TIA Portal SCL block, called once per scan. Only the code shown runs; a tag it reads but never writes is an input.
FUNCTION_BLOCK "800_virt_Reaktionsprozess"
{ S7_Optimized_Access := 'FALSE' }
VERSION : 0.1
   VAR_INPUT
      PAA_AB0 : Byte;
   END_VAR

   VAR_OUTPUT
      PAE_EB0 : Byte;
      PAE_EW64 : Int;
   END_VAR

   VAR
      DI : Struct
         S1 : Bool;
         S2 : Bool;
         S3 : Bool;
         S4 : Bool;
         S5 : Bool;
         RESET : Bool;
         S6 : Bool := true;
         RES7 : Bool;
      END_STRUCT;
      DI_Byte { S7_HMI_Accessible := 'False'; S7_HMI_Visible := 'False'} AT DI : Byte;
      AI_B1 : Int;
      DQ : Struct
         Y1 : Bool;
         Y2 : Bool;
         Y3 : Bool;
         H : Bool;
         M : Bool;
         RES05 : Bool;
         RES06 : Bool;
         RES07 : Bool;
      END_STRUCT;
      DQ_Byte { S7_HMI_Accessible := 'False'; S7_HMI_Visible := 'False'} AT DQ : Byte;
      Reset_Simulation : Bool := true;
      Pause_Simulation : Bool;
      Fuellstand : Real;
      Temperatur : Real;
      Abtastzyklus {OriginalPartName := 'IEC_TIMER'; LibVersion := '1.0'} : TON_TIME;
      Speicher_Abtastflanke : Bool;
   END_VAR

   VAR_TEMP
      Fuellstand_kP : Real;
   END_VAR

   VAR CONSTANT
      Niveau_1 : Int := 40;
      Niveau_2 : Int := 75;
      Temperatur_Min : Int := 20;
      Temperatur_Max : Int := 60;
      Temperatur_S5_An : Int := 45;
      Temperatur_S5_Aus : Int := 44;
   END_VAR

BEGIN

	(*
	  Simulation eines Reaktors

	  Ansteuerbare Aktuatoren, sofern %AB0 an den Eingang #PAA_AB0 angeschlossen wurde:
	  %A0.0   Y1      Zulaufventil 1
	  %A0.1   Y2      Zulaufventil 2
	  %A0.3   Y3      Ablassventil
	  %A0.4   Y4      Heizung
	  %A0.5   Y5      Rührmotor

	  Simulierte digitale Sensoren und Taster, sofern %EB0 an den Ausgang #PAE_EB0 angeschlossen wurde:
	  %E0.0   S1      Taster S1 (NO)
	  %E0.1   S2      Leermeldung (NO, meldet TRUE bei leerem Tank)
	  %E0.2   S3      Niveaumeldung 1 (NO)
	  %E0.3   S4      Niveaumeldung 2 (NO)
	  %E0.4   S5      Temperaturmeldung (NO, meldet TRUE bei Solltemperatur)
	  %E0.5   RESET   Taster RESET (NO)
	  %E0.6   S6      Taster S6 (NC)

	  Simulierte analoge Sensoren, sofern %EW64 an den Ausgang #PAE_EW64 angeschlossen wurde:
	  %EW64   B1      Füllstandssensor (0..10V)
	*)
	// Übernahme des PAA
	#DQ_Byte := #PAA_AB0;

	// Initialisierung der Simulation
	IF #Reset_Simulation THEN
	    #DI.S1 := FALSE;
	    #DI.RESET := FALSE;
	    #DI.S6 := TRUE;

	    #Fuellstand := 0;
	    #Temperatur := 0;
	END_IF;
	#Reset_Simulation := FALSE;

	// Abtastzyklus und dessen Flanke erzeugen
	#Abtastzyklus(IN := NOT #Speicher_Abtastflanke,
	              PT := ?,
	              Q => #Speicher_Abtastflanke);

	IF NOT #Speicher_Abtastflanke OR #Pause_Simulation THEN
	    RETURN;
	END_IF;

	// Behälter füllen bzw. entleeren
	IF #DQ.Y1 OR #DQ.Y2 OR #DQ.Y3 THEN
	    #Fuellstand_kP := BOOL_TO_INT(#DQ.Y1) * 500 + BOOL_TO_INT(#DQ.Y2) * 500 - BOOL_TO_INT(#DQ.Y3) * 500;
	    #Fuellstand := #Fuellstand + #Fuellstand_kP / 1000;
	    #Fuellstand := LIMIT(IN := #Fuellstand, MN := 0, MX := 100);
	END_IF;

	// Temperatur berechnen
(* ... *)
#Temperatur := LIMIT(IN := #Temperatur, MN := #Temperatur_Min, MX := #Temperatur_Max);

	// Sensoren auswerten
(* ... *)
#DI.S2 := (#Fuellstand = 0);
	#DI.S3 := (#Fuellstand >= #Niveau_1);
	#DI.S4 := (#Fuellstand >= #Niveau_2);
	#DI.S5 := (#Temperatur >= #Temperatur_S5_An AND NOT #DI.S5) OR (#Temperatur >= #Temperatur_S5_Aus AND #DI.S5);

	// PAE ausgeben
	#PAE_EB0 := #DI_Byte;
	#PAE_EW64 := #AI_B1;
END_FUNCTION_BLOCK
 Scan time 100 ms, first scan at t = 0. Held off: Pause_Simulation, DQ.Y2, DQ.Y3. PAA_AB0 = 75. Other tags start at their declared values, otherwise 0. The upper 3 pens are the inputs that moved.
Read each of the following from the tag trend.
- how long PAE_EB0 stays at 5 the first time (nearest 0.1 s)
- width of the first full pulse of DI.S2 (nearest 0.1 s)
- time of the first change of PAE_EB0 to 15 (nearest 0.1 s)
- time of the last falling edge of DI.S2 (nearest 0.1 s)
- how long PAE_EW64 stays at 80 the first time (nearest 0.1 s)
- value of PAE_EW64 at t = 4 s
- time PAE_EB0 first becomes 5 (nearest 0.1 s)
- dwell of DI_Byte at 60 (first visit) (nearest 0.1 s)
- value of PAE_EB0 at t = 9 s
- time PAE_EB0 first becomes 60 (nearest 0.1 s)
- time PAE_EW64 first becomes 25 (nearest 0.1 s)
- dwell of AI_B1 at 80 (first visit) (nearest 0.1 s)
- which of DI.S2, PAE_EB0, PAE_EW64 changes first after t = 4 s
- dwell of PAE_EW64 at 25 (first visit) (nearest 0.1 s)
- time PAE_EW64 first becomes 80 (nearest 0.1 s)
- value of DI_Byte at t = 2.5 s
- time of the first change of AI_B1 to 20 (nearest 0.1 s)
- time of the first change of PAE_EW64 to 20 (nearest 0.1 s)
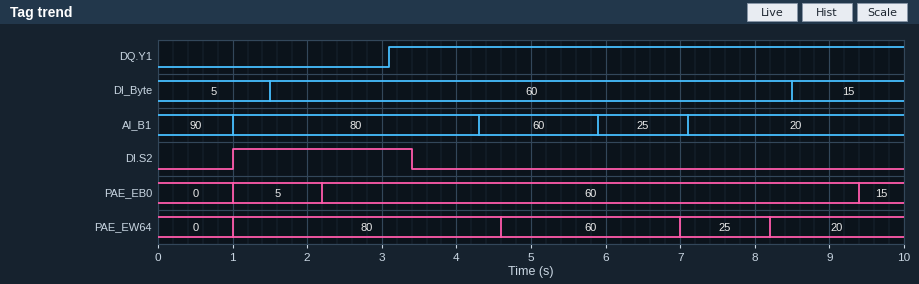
1.2 s
2.4 s
9.4 s
3.4 s
3.6 s
80
1.0 s
7.0 s
60
2.2 s
7.0 s
3.3 s
PAE_EW64
1.2 s
1.0 s
60
7.1 s
8.2 s
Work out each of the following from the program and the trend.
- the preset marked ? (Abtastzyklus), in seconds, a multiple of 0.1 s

1.0 s
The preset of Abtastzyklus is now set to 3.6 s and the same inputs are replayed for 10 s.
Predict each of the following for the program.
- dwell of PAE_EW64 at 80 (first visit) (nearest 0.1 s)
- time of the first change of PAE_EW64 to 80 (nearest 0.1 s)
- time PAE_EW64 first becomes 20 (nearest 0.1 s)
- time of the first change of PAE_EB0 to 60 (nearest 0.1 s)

3.8 s
3.6 s
7.4 s
3.6 s
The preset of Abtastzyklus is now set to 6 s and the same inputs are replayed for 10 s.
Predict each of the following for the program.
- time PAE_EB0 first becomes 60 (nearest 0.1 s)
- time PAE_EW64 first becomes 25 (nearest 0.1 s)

6.0 s
6.0 s
